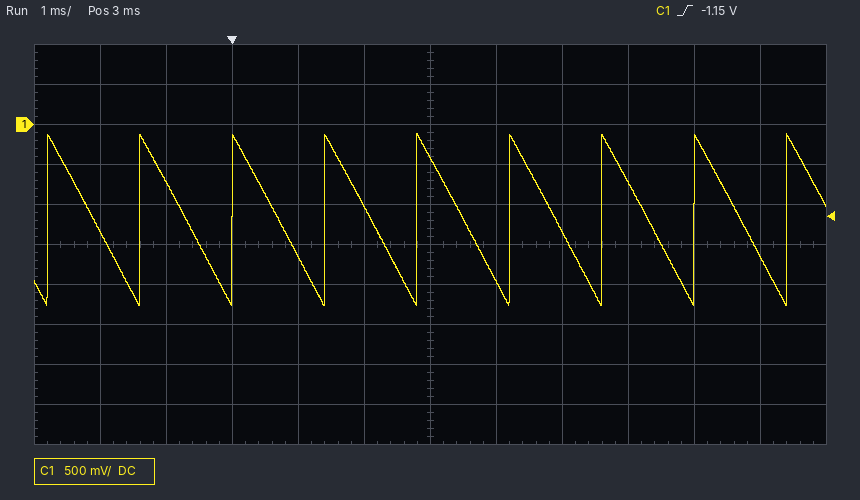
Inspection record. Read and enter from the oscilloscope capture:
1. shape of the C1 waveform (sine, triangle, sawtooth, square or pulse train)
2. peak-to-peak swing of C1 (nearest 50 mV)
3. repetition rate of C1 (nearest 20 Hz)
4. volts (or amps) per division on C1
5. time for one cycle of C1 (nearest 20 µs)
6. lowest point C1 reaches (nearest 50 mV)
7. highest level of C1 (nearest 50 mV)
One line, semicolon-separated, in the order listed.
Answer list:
sawtooth; 2.15 V; 720 Hz; 500 mV; 1.40 ms; -2.25 V; -100 mV
